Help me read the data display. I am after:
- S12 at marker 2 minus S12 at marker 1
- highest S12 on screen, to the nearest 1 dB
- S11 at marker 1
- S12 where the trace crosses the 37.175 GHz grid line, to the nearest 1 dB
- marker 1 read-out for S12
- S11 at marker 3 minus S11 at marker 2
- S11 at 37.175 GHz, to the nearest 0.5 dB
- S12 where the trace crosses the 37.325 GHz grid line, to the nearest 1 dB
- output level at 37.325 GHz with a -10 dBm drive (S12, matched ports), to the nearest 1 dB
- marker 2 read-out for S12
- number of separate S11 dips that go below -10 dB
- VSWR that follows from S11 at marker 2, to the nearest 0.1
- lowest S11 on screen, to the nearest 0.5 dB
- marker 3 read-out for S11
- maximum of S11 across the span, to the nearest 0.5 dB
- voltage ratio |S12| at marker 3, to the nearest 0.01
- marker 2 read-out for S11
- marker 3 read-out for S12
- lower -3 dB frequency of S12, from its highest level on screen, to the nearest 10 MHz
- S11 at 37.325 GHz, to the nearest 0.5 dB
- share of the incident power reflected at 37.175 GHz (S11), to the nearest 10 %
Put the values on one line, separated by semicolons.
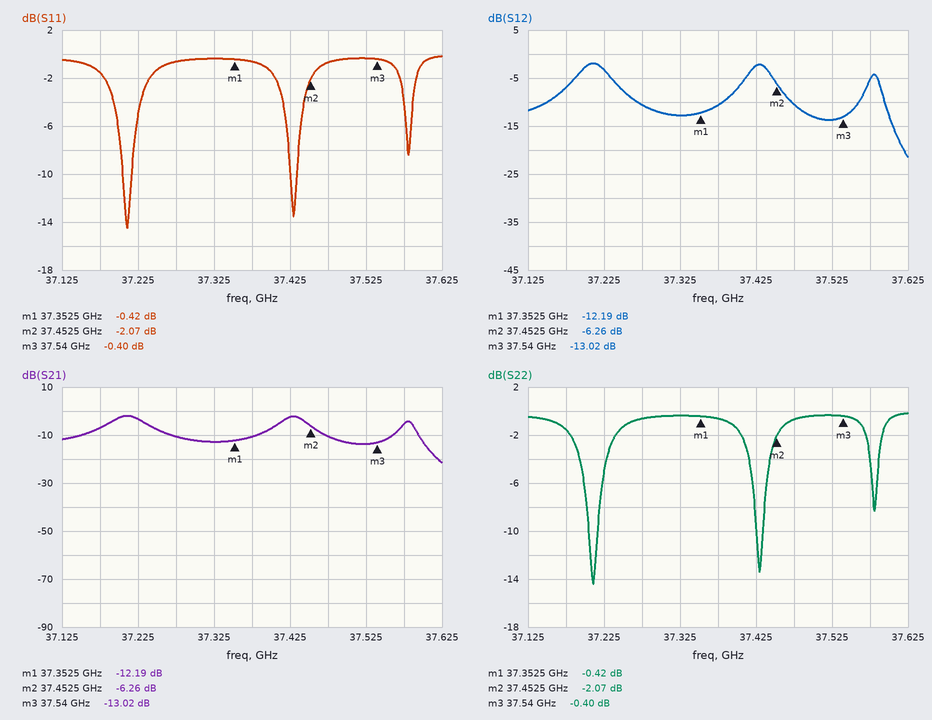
5.93 dB; -2 dB; -0.42 dB; -7 dB; -12.19 dB; 1.67 dB; -1.5 dB; -13 dB; -23 dBm; -6.26 dB; 2; 8.4; -14.5 dB; -0.40 dB; 0.0 dB; 0.22; -2.07 dB; -13.02 dB; 37.19 GHz; -0.5 dB; 70 %
